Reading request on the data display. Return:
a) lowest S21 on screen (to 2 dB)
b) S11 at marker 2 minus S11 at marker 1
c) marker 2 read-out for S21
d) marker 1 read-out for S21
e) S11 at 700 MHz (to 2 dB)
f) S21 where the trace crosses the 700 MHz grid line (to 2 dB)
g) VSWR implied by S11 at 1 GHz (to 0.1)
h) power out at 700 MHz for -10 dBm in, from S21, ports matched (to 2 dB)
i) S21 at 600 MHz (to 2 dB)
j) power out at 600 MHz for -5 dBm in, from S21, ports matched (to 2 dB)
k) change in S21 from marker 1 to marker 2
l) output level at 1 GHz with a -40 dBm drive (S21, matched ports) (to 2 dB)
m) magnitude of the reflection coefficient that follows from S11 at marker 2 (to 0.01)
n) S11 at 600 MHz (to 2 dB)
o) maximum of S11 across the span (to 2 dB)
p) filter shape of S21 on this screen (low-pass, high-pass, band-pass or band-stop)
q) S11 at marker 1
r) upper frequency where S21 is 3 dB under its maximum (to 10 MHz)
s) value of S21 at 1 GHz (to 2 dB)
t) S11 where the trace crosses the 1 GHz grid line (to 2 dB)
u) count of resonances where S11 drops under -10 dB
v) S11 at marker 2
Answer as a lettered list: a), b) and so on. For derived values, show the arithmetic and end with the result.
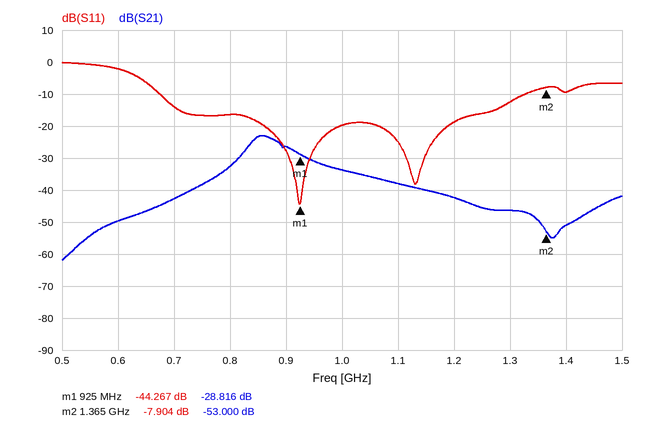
a) -62 dB
b) -7.904 − (-44.267) = 36.363 dB
c) -53.000 dB
d) -28.816 dB
e) -14 dB
f) -42 dB
g) |Γ| = 10^(-20/20) = 0.1000; VSWR = (1 + 0.1000)/(1 − 0.1000) ≈ 1.2
h) -10 dBm + (-42 dB) = -52 dBm
i) -50 dB
j) -5 dBm + (-50 dB) = -54 dBm
k) -53 − (-28.816) = -24.184 dB
l) -40 dBm + (-34 dB) = -74 dBm
m) 10^(-7.904/20) ≈ 0.40
n) -2 dB
o) 0 dB
p) band-pass
q) -44.267 dB
r) 890 MHz
s) -34 dB
t) -20 dB
u) 2
v) -7.904 dB
